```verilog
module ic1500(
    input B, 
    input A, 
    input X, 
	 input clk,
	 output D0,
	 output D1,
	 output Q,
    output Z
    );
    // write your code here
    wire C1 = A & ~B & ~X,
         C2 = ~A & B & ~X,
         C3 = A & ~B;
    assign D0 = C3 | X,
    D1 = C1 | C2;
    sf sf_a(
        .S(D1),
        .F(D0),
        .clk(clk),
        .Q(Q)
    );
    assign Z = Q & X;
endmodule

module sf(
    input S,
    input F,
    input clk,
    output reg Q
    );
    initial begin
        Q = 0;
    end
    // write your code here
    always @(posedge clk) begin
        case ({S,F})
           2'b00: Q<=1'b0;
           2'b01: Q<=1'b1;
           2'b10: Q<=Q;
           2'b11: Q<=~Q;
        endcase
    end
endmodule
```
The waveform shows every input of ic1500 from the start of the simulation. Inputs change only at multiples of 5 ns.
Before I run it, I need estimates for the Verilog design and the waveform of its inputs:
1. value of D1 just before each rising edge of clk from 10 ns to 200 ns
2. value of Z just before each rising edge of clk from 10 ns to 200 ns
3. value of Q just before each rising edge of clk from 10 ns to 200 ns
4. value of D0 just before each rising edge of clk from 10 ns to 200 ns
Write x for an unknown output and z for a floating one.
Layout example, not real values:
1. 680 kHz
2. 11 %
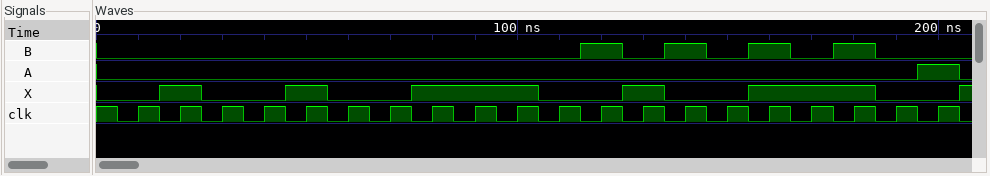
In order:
1. 0 0 0 0 0 0 0 0 0 0 0 1 0 1 0 0 0 0 0 1
2. 0 0 0 0 0 0 0 0 1 1 0 0 0 0 0 0 1 1 0 0
3. 0 0 1 0 0 1 0 0 1 1 1 0 0 1 1 0 1 1 1 0
4. 0 1 0 0 1 0 0 1 1 1 0 0 1 0 0 1 1 1 0 1
